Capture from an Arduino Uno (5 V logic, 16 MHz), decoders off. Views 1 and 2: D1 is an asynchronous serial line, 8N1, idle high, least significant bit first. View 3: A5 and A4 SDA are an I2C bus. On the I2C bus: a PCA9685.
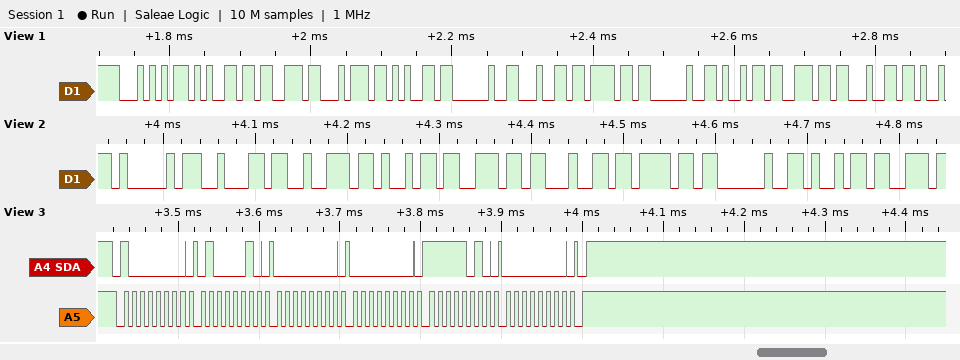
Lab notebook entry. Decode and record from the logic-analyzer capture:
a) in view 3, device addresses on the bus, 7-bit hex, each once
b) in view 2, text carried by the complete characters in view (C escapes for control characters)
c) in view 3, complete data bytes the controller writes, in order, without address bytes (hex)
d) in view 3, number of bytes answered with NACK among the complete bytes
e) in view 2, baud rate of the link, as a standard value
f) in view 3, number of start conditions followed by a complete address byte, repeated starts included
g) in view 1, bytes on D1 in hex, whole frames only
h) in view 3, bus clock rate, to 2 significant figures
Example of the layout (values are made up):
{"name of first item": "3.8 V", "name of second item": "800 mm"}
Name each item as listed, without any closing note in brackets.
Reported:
{"in view 3, device addresses on the bus, 7-bit hex, each once": "0x40", "in view 2, text carried by the complete characters in view": "\"Abrindo i\"", "in view 3, complete data bytes the controller writes, in order, without address bytes": "42 00 00 FA 00", "in view 3, number of bytes answered with NACK among the complete bytes": "0", "in view 2, baud rate of the link, as a standard value": "115200 baud", "in view 3, number of start conditions followed by a complete address byte, repeated starts included": "1", "in view 1, bytes on D1 in hex, whole frames only": "54 65 73 74 65 20 64 6F 20 69 6E 64", "in view 3, bus clock rate, to 2 significant figures": "100 kHz"}
